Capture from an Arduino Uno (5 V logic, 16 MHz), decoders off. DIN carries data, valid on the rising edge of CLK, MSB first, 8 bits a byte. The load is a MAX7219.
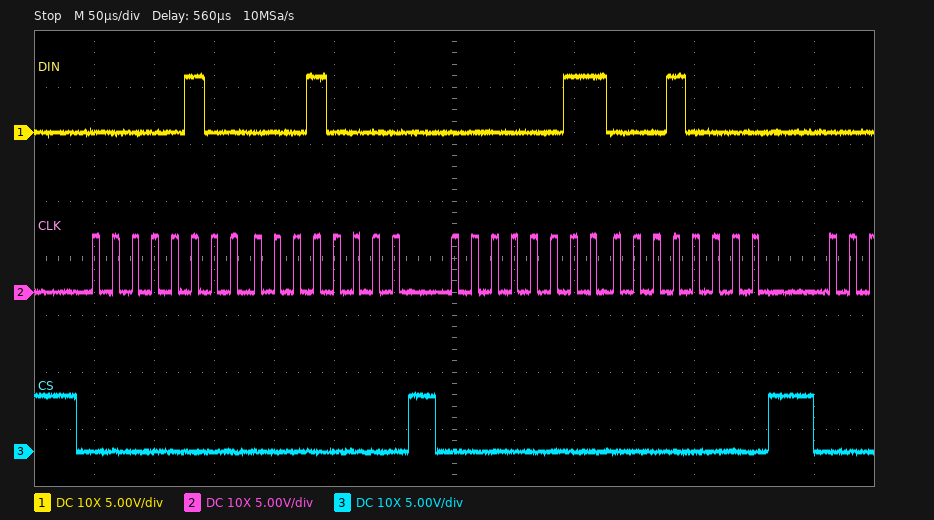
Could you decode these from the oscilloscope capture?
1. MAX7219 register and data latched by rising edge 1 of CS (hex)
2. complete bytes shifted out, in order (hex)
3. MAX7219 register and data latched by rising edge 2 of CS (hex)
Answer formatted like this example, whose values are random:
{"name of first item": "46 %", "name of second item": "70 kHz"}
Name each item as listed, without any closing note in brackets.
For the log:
{"MAX7219 register and data latched by rising edge 1 of CS": "register 0x4, data 0x10", "complete bytes shifted out, in order": "0x04 0x10 0x03 0x10", "MAX7219 register and data latched by rising edge 2 of CS": "register 0x3, data 0x10"}
